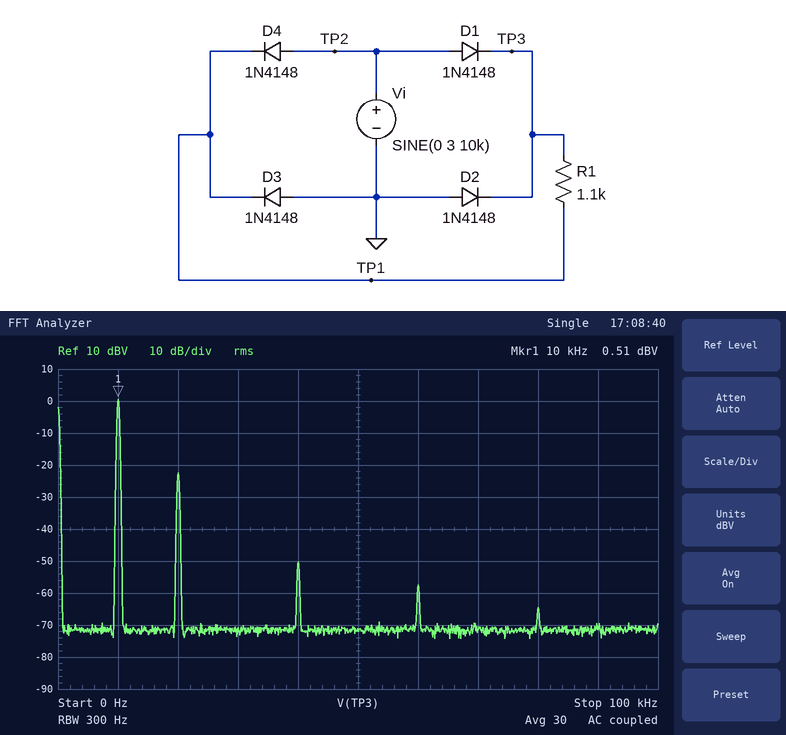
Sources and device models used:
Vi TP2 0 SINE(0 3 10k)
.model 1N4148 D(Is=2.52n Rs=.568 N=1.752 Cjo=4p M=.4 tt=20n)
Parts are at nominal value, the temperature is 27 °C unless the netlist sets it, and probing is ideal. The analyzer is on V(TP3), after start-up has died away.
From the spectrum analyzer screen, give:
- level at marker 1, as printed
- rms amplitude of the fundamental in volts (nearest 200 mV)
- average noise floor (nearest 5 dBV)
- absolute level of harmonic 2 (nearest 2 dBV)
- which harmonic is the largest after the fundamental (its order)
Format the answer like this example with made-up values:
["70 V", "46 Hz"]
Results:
["0.51 dBV", "1.0 V", "-70 dBV", "-22 dBV", "2"]
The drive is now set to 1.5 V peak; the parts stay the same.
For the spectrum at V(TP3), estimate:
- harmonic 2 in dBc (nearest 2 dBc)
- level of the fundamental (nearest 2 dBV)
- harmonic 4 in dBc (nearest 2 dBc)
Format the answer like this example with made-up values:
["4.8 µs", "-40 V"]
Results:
["-26 dBc", "-6 dBV", "-48 dBc"]
